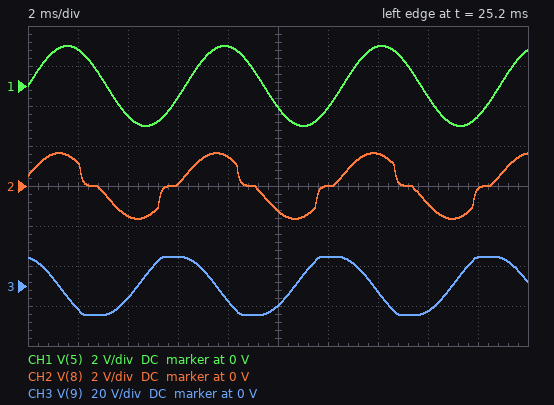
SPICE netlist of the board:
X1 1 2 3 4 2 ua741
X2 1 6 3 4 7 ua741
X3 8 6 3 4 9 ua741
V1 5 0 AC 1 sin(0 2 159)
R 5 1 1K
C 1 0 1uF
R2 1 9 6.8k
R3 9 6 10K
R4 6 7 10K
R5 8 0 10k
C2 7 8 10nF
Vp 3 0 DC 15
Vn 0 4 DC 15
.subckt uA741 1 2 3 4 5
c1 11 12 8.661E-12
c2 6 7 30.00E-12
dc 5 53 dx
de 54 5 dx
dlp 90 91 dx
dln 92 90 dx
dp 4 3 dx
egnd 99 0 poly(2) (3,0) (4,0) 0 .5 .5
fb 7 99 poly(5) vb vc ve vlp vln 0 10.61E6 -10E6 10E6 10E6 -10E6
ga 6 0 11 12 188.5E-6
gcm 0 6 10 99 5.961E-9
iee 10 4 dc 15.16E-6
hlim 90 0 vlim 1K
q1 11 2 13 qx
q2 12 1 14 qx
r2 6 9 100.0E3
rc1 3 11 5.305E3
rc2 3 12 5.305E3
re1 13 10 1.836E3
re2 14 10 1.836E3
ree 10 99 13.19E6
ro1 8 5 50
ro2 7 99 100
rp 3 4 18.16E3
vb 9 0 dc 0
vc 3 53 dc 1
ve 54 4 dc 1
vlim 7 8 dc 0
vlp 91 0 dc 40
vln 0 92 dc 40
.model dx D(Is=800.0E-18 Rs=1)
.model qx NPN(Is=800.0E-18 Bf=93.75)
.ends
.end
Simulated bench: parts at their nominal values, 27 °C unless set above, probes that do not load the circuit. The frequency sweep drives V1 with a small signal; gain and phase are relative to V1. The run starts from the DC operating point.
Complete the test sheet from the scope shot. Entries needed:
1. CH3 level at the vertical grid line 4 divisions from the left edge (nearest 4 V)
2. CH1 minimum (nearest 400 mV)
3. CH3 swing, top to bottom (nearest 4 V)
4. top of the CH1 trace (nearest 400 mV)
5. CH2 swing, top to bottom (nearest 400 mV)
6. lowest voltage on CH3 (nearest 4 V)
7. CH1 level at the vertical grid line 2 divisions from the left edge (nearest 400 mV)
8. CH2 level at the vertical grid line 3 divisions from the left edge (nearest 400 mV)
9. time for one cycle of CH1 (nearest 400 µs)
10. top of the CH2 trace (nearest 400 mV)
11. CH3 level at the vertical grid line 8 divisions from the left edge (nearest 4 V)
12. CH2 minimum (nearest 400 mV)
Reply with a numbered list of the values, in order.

1. -8 V
2. -2.0 V
3. 28 V
4. 2.0 V
5. 3.2 V
6. -16 V
7. -1.6 V
8. 0 V
9. 6.4 ms
10. 1.6 V
11. -12 V
12. -1.6 V
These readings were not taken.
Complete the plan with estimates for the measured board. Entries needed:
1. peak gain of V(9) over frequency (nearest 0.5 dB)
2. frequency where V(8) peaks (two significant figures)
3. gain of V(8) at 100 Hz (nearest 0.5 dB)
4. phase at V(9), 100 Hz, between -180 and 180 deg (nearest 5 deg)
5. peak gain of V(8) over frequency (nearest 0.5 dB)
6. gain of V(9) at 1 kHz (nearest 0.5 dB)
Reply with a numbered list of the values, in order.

1. 19.0 dB
2. 190 Hz
3. -6.0 dB
4. 145 deg
5. 0 dB
6. -10.5 dB
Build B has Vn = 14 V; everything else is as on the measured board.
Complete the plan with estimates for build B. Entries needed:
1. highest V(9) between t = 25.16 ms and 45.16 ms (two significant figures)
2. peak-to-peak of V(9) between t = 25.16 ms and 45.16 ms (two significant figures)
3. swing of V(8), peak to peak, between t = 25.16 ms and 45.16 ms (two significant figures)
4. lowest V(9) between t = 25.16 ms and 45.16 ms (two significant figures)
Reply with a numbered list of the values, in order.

1. 14 V
2. 27 V
3. 3.2 V
4. -14 V
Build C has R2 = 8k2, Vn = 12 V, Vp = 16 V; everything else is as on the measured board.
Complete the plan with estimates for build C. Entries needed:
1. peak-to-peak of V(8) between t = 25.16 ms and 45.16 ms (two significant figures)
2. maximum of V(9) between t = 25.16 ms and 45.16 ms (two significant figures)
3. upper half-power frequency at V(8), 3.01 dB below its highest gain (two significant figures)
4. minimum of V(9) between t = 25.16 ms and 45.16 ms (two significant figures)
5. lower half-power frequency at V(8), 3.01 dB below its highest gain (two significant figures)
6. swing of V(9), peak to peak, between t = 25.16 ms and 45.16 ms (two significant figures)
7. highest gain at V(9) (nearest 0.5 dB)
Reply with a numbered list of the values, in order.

1. 3.2 V
2. 12 V
3. 270 Hz
4. -12 V
5. 110 Hz
6. 23 V
7. 20.0 dB
